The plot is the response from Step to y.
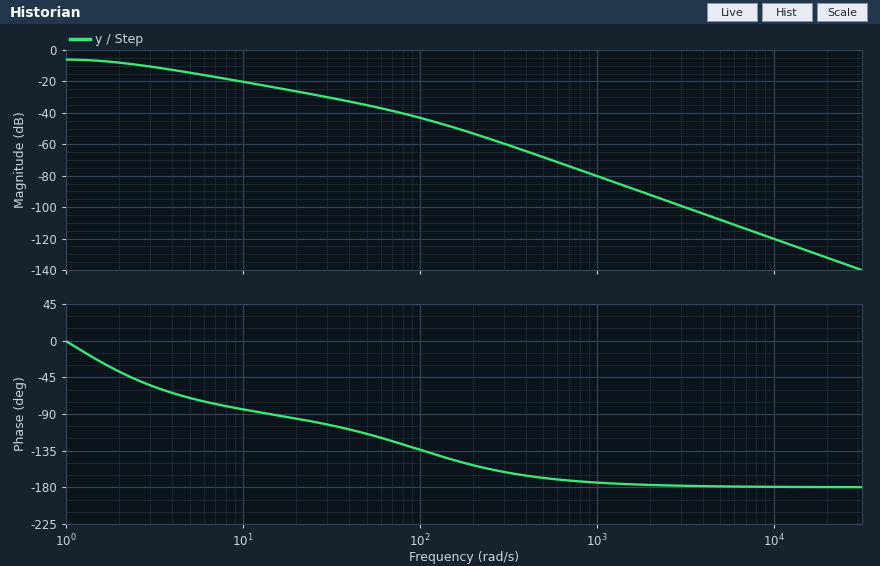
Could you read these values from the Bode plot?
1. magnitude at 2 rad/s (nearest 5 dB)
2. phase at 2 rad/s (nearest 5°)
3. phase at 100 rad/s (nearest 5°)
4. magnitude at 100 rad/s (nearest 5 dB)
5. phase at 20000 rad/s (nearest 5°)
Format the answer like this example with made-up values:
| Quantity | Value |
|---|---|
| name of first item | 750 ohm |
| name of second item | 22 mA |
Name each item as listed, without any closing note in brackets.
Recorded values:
| Quantity | Value |
|---|---|
| magnitude at 2 rad/s | -10 dB |
| phase at 2 rad/s | -40° |
| phase at 100 rad/s | -135° |
| magnitude at 100 rad/s | -45 dB |
| phase at 20000 rad/s | -180° |
